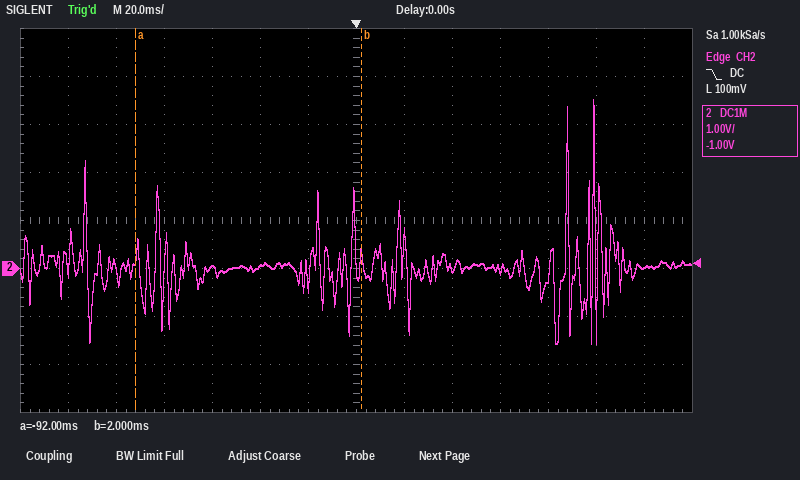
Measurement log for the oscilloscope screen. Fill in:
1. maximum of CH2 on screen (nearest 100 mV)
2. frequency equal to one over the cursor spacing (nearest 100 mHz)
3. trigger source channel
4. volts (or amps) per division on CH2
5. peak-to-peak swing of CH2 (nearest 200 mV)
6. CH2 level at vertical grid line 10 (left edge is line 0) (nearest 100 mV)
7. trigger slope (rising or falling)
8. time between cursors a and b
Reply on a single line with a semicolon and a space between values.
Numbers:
3.5 V; 10.6 Hz; CH2; 1 V; 5.0 V; 0.0 V; falling; 94 ms
